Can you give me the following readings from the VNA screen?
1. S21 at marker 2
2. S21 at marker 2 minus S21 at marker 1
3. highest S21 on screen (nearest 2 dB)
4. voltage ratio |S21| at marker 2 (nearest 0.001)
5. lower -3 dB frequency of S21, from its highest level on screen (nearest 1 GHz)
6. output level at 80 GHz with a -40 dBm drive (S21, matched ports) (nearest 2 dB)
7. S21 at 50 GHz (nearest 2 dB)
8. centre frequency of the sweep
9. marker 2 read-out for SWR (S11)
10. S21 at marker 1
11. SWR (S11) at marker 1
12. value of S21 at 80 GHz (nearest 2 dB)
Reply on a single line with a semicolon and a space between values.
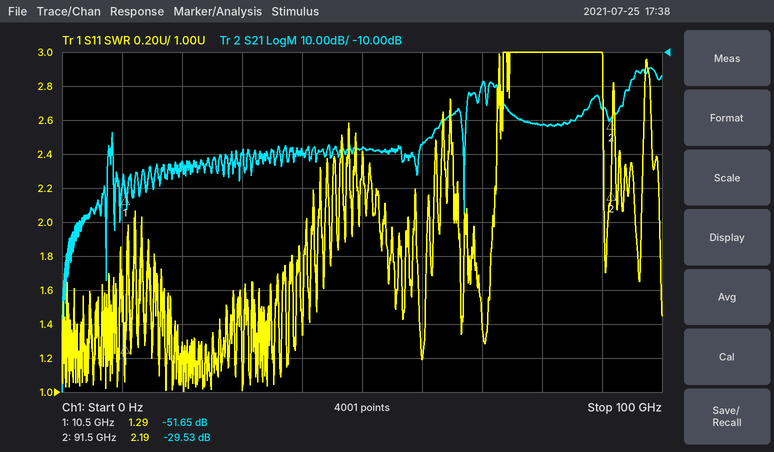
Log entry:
-29.53 dB; 22.12 dB; -14 dB; 0.033; 95 GHz; -72 dBm; -38 dB; 50 GHz; 2.19; -51.65 dB; 1.29; -32 dB
